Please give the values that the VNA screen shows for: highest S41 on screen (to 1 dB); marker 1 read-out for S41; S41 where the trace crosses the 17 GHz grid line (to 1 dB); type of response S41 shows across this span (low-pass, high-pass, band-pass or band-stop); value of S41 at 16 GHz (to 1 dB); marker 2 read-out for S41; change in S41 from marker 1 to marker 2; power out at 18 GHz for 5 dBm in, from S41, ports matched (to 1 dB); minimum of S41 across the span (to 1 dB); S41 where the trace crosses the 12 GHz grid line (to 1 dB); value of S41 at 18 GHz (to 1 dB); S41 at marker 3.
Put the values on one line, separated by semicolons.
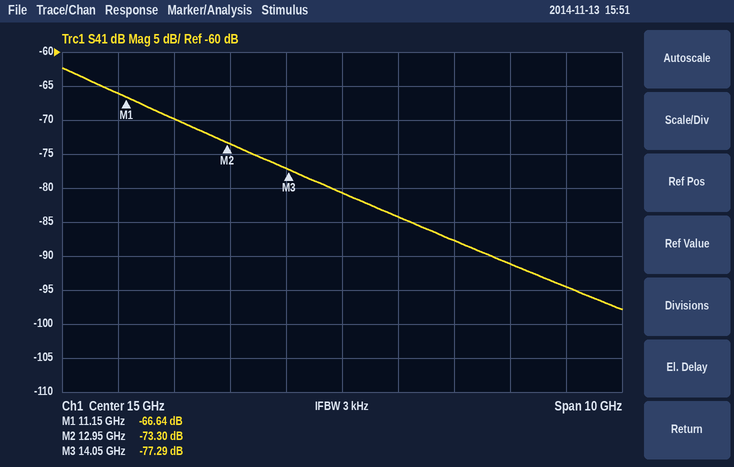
-62 dB; -66.64 dB; -88 dB; low-pass; -84 dB; -73.30 dB; -6.66 dB; -86 dBm; -98 dB; -70 dB; -91 dB; -77.29 dB
